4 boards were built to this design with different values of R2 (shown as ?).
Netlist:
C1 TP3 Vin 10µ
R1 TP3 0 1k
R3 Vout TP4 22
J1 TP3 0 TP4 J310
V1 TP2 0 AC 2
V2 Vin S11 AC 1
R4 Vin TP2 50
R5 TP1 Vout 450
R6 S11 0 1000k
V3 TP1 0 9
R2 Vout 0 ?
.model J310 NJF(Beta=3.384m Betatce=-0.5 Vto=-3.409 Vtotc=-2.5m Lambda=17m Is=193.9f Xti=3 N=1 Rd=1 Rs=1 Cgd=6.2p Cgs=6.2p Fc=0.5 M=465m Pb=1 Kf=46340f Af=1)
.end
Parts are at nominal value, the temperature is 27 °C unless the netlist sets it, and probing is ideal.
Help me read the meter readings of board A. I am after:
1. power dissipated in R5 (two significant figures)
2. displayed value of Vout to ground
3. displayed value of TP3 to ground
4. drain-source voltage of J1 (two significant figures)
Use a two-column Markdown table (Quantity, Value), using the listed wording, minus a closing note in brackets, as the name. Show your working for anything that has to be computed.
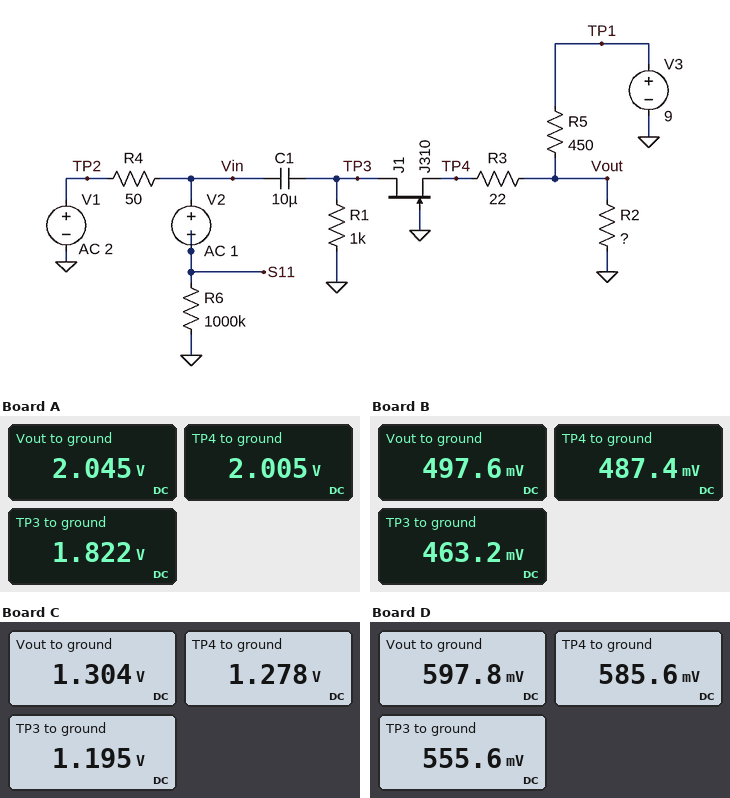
| Quantity | Value |
|---|---|
| power dissipated in R5 | (9 V - 2.045 V)^2 / 450 Ω = 110 mW |
| displayed value of Vout to ground | 2.045 V |
| displayed value of TP3 to ground | 1.822 V |
| drain-source voltage of J1 | 1.822 V - 2.005 V = -180 mV |
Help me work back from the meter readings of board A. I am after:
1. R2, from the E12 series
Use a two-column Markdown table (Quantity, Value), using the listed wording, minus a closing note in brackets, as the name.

| Quantity | Value |
|---|---|
| R2, from the E12 series | 150 Ω |
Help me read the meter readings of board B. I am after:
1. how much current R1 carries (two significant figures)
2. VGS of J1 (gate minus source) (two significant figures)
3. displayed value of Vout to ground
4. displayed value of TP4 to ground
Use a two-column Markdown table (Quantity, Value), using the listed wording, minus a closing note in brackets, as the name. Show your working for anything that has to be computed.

| Quantity | Value |
|---|---|
| how much current R1 carries | (463.2 mV) / 1 kΩ = 460 µA |
| VGS of J1 (gate minus source) | 0 V - 487.4 mV = -490 mV |
| displayed value of Vout to ground | 497.6 mV |
| displayed value of TP4 to ground | 487.4 mV |
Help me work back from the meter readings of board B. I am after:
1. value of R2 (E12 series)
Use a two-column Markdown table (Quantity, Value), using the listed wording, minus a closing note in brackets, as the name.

| Quantity | Value |
|---|---|
| value of R2 | 27 Ω |
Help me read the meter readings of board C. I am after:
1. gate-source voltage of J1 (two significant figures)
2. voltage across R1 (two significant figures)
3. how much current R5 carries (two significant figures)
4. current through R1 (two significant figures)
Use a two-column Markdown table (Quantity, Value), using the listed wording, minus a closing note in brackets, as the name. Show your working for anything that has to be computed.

| Quantity | Value |
|---|---|
| gate-source voltage of J1 | 0 V - 1.278 V = -1.3 V |
| voltage across R1 | 1.195 V = 1.2 V |
| how much current R5 carries | (9 V - 1.304 V) / 450 Ω = 17 mA |
| current through R1 | (1.195 V) / 1 kΩ = 1.2 mA |
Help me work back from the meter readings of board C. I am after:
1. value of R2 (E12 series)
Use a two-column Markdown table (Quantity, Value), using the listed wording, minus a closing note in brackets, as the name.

| Quantity | Value |
|---|---|
| value of R2 | 82 Ω |
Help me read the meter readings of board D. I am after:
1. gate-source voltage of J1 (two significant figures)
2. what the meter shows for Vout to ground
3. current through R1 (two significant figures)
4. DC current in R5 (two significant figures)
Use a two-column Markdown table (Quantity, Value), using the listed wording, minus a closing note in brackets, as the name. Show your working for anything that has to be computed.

| Quantity | Value |
|---|---|
| gate-source voltage of J1 | 0 V - 585.6 mV = -590 mV |
| what the meter shows for Vout to ground | 597.8 mV |
| current through R1 | (555.6 mV) / 1 kΩ = 560 µA |
| DC current in R5 | (9 V - 597.8 mV) / 450 Ω = 19 mA |
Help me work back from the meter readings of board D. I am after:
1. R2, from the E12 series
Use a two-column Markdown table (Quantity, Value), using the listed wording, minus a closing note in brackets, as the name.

| Quantity | Value |
|---|---|
| R2, from the E12 series | 33 Ω |
